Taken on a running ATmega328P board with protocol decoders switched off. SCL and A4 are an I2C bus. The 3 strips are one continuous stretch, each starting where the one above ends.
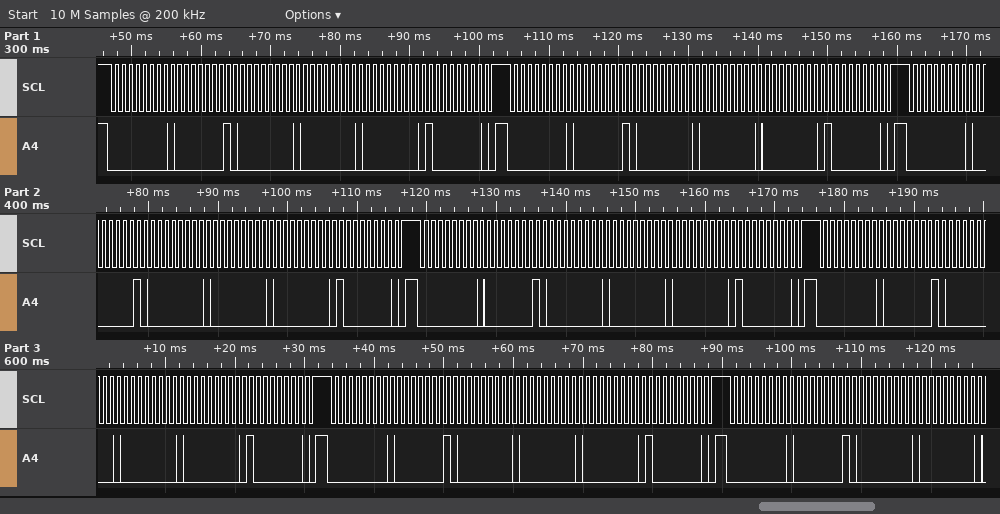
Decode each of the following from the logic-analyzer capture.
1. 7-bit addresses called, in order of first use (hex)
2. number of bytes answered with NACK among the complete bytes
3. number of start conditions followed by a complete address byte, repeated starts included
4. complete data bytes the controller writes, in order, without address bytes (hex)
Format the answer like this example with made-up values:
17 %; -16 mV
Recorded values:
0x00; 0; 7; 01 00 00 00 80 01 00 00 00 80 01 00 00 00 80 01 00 00 00 80 01 00 00 00 80 01 00 00 00 80 01 00 00
